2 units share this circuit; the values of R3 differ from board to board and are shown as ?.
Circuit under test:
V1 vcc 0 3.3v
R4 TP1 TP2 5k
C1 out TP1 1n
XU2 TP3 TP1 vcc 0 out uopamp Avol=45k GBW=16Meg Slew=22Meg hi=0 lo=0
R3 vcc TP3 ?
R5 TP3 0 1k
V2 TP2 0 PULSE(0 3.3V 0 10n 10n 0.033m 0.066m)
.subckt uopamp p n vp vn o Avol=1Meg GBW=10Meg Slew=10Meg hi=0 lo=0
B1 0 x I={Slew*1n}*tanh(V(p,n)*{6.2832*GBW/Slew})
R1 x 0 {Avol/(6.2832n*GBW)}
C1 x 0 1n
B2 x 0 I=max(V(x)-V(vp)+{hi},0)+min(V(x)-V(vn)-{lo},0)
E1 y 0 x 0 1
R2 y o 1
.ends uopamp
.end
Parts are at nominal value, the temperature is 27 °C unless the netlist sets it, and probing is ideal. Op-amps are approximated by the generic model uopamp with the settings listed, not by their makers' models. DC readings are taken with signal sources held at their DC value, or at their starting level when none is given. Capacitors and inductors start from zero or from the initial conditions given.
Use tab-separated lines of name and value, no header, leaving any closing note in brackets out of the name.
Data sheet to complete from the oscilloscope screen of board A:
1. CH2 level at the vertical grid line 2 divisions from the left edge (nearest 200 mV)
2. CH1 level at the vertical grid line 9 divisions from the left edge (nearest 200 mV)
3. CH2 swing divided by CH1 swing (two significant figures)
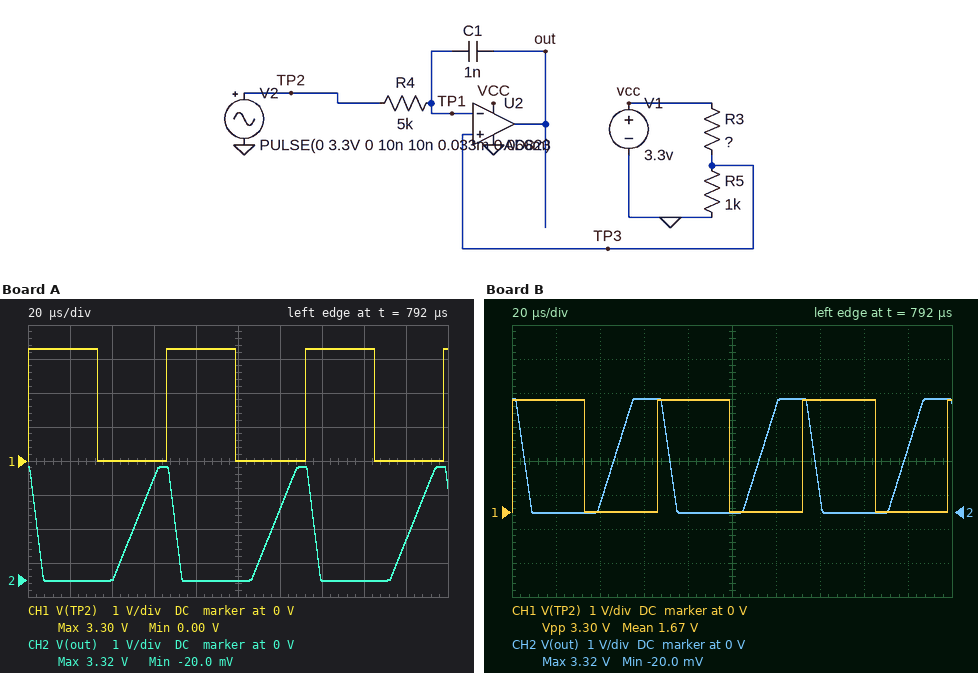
CH2 level at the vertical grid line 2 divisions from the left edge	0 V
CH1 level at the vertical grid line 9 divisions from the left edge	0 V
CH2 swing divided by CH1 swing	1.0
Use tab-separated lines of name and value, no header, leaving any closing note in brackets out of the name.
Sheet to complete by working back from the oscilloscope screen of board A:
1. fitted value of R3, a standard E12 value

fitted value of R3, a standard E12 value	3.3 kΩ
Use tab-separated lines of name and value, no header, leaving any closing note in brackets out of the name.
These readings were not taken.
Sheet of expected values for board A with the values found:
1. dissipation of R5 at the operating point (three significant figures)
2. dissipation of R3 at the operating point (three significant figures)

dissipation of R5 at the operating point	589 µW
dissipation of R3 at the operating point	1.94 mW
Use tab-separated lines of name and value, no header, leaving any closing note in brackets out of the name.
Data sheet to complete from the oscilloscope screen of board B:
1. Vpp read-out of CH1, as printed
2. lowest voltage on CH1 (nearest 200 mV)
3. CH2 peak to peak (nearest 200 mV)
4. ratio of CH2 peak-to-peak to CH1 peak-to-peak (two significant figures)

Vpp read-out of CH1, as printed	3.30 V
lowest voltage on CH1	0 V
CH2 peak to peak	3.4 V
ratio of CH2 peak-to-peak to CH1 peak-to-peak	1.0
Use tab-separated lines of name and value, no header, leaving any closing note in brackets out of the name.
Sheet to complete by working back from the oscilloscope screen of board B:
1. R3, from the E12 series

R3, from the E12 series	2.2 kΩ
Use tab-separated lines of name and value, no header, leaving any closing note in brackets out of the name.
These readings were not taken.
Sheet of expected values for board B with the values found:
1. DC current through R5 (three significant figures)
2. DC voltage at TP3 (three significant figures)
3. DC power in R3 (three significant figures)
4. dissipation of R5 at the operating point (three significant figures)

DC current through R5	1.03 mA
DC voltage at TP3	1.03 V
DC power in R3	2.34 mW
dissipation of R5 at the operating point	1.06 mW
